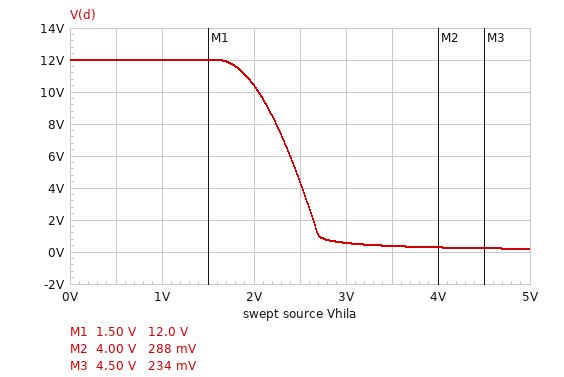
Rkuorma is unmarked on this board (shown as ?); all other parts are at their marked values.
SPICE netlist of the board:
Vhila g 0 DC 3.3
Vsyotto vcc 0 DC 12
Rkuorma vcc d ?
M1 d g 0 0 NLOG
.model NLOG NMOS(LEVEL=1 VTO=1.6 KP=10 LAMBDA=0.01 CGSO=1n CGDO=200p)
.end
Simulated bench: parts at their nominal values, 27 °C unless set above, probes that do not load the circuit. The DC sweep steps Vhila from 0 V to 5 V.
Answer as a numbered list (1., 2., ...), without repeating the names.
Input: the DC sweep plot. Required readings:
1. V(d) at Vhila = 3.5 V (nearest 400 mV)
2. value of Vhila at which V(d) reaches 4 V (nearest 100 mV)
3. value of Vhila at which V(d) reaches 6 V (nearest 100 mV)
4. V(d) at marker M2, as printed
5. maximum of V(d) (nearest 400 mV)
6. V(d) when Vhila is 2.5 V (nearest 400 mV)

1. 400 mV
2. 2.5 V
3. 2.4 V
4. 288 mV
5. 12.0 V
6. 4.4 V
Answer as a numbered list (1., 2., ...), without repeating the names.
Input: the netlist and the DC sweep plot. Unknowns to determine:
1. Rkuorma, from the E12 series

1. 1.8 Ω
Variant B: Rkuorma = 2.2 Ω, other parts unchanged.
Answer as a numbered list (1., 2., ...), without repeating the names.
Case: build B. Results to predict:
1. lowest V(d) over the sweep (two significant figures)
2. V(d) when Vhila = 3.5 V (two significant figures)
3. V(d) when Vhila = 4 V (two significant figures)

1. 160 mV
2. 300 mV
3. 230 mV
